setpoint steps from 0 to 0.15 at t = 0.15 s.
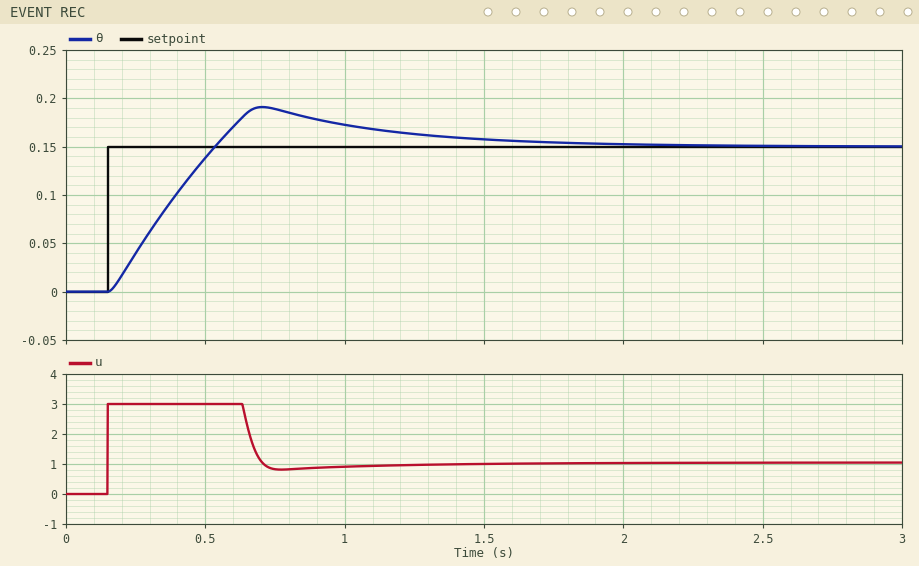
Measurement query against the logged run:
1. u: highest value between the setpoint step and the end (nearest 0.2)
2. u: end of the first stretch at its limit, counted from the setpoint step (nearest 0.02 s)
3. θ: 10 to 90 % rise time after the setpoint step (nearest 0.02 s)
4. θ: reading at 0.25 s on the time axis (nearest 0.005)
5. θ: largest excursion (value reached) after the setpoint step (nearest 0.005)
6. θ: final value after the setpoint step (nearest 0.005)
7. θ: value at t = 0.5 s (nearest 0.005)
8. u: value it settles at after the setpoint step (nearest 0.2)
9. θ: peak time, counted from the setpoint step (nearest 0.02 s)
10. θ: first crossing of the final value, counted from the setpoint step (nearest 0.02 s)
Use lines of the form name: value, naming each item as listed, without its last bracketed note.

u: highest value between the setpoint step and the end: 3.0
u: end of the first stretch at its limit, counted from the setpoint step: 0.48 s
θ: 10 to 90 % rise time after the setpoint step: 0.30 s
θ: reading at 0.25 s on the time axis: 0.040
θ: largest excursion (value reached) after the setpoint step: 0.190
θ: final value after the setpoint step: 0.150
θ: value at t = 0.5 s: 0.140
u: value it settles at after the setpoint step: 1.0
θ: peak time, counted from the setpoint step: 0.56 s
θ: first crossing of the final value, counted from the setpoint step: 0.38 s
